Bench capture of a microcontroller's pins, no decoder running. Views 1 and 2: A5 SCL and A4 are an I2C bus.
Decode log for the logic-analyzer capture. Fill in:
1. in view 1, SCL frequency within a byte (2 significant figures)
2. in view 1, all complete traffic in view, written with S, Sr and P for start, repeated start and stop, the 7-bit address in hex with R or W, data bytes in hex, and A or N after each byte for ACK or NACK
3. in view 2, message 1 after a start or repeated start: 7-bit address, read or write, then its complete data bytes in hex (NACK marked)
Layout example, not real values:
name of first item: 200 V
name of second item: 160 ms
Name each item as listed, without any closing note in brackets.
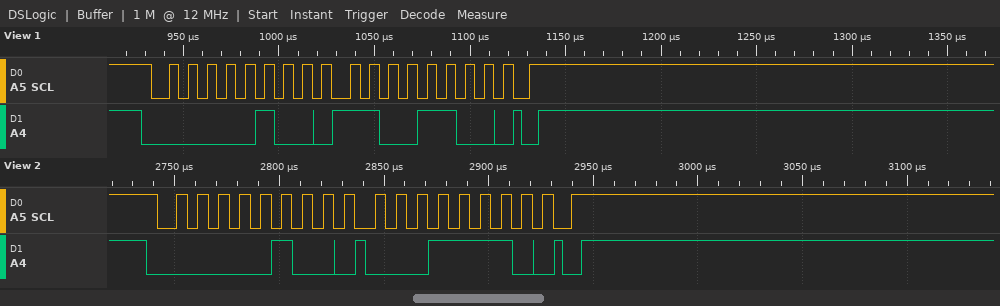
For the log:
in view 1, SCL frequency within a byte: 100 kHz
in view 1, all complete traffic in view, written with S, Sr and P for start, repeated start and stop, the 7-bit address in hex with R or W, data bytes in hex, and A or N after each byte for ACK or NACK: S 02W A CC A P
in view 2, message 1 after a start or repeated start: 7-bit address, read or write, then its complete data bytes in hex: 0x02 write: 1E
